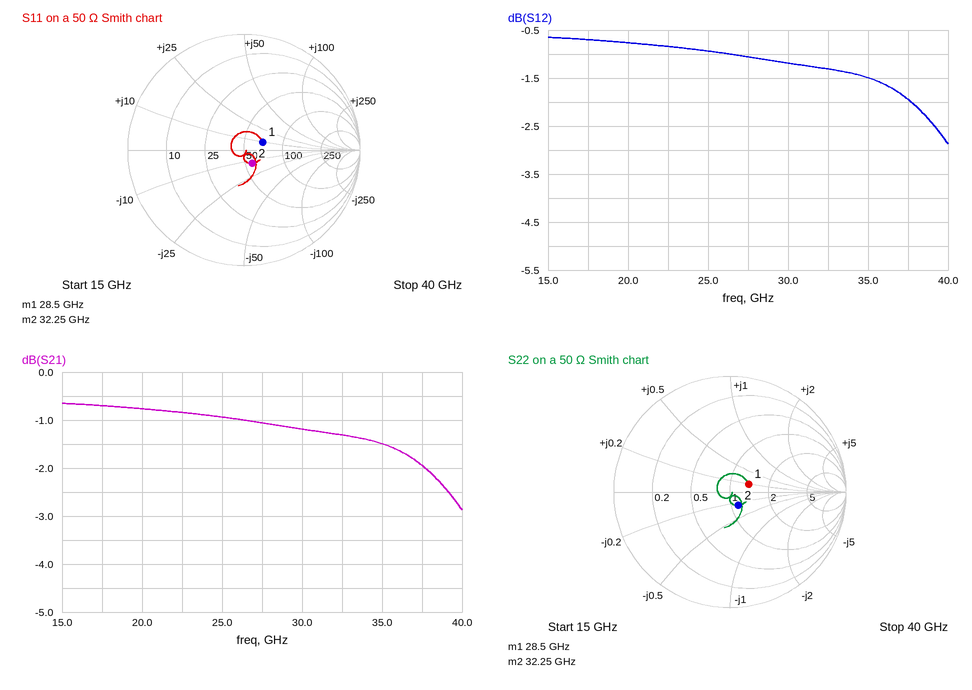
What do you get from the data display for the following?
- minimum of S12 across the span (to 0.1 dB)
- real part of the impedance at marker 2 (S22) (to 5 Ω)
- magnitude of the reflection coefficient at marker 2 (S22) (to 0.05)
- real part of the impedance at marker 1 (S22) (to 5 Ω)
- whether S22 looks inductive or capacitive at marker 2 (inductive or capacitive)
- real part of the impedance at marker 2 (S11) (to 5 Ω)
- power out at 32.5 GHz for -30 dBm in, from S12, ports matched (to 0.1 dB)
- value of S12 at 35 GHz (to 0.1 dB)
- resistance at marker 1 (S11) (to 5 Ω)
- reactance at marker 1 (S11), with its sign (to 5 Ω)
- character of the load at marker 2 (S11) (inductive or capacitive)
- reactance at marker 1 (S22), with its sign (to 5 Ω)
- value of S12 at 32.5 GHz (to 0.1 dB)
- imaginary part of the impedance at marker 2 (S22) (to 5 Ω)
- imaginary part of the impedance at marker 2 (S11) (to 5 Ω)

-2.9 dB
55 Ω
0.15
70 Ω
capacitive
55 Ω
-31.3 dBm
-1.5 dB
70 Ω
+10 Ω
capacitive
+10 Ω
-1.3 dB
-15 Ω
-15 Ω
